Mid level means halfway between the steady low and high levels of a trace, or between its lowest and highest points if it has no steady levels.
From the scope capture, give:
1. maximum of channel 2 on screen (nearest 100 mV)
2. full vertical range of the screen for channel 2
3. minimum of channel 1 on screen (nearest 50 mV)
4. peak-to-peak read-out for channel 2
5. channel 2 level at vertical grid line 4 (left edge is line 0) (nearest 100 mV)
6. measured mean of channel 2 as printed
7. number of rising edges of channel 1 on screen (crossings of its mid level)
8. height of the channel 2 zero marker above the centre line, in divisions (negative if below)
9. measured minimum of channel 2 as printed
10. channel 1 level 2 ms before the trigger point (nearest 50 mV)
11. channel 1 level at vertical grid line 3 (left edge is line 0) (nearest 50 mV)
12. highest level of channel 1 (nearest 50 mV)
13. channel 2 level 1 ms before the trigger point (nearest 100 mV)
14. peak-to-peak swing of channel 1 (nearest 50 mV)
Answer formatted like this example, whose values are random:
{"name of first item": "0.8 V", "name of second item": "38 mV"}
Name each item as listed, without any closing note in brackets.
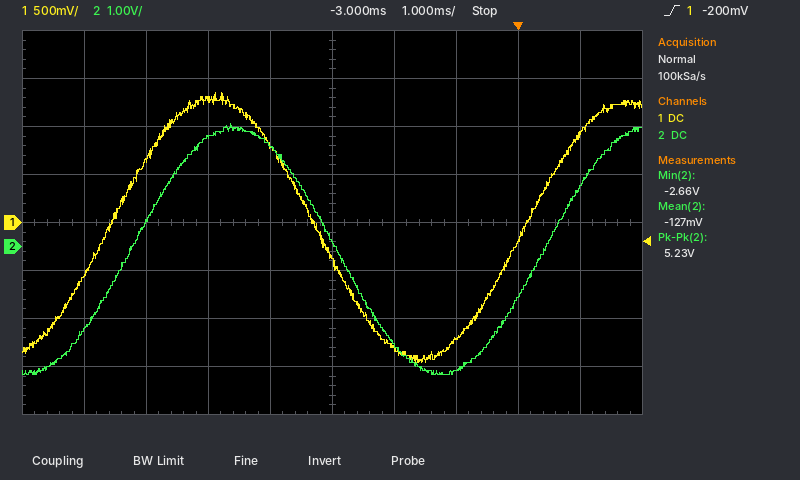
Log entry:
{"maximum of channel 2 on screen": "2.6 V", "full vertical range of the screen for channel 2": "8 V", "minimum of channel 1 on screen": "-1.45 V", "peak-to-peak read-out for channel 2": "5.23 V", "channel 2 level at vertical grid line 4 (left edge is line 0)": "2.1 V", "measured mean of channel 2 as printed": "-127 mV", "number of rising edges of channel 1 on screen": "2", "height of the channel 2 zero marker above the centre line, in divisions": "-0.5 div", "measured minimum of channel 2 as printed": "-2.66 V", "channel 1 level 2 ms before the trigger point": "-1.30 V", "channel 1 level at vertical grid line 3 (left edge is line 0)": "1.30 V", "highest level of channel 1": "1.35 V", "channel 2 level 1 ms before the trigger point": "-2.6 V", "peak-to-peak swing of channel 1": "2.80 V"}
